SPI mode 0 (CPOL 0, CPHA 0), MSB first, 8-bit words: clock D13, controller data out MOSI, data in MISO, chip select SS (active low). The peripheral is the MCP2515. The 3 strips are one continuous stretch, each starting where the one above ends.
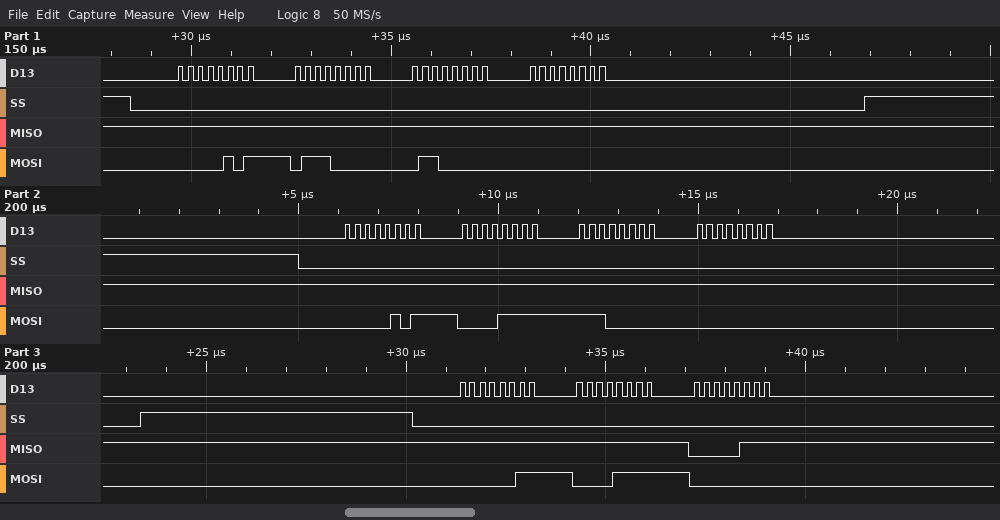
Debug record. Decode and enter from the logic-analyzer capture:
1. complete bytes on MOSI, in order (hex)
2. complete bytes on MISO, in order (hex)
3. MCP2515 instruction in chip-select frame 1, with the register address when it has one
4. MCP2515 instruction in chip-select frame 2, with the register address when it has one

05 70 60 00 05 0F E0 00 03 0F 00
FF FF FF FF FF FF FF FF FF FF 07
BIT MODIFY 0x70
BIT MODIFY 0x0F
